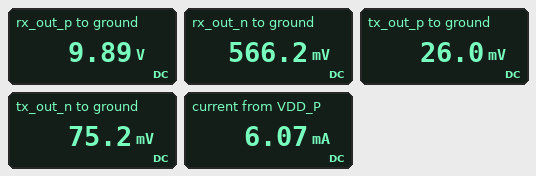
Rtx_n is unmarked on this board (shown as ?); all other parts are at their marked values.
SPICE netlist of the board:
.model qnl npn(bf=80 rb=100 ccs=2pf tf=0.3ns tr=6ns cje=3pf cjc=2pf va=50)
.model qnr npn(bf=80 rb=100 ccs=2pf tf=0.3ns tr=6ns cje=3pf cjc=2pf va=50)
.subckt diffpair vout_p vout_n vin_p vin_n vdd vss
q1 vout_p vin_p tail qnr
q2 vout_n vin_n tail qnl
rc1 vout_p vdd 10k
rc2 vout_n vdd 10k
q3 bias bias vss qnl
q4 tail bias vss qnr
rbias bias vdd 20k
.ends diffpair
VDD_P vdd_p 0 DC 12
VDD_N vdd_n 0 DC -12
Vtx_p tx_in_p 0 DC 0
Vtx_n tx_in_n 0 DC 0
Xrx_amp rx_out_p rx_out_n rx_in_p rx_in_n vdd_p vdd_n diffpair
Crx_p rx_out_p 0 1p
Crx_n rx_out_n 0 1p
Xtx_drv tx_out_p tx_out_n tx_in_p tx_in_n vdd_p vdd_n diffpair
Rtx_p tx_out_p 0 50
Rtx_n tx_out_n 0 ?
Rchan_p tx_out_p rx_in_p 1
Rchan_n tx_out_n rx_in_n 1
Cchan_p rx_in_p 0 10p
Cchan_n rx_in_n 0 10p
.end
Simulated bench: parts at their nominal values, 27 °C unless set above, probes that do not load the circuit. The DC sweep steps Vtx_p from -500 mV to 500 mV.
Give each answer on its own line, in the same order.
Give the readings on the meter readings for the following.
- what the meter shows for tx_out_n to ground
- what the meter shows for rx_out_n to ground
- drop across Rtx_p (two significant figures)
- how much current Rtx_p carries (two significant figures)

75.2 mV
566.2 mV
26 mV
520 µA
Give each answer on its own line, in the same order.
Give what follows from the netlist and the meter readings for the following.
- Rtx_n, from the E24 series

150 Ω
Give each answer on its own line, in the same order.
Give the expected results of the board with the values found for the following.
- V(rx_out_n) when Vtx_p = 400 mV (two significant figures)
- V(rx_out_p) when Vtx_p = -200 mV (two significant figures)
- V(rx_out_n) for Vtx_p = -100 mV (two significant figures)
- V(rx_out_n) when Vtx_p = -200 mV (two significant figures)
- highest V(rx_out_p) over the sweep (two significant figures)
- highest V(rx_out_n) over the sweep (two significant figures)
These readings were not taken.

-560 mV
-610 mV
11 V
11 V
12 V
11 V
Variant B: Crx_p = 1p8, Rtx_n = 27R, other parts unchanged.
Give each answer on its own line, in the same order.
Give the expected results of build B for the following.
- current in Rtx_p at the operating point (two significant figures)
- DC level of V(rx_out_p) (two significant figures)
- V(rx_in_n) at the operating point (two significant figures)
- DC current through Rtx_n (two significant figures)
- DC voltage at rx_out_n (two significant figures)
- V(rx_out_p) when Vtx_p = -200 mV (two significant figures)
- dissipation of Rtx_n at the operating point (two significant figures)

510 µA
3.9 V
14 mV
520 µA
6.5 V
-170 mV
7.2 µW
